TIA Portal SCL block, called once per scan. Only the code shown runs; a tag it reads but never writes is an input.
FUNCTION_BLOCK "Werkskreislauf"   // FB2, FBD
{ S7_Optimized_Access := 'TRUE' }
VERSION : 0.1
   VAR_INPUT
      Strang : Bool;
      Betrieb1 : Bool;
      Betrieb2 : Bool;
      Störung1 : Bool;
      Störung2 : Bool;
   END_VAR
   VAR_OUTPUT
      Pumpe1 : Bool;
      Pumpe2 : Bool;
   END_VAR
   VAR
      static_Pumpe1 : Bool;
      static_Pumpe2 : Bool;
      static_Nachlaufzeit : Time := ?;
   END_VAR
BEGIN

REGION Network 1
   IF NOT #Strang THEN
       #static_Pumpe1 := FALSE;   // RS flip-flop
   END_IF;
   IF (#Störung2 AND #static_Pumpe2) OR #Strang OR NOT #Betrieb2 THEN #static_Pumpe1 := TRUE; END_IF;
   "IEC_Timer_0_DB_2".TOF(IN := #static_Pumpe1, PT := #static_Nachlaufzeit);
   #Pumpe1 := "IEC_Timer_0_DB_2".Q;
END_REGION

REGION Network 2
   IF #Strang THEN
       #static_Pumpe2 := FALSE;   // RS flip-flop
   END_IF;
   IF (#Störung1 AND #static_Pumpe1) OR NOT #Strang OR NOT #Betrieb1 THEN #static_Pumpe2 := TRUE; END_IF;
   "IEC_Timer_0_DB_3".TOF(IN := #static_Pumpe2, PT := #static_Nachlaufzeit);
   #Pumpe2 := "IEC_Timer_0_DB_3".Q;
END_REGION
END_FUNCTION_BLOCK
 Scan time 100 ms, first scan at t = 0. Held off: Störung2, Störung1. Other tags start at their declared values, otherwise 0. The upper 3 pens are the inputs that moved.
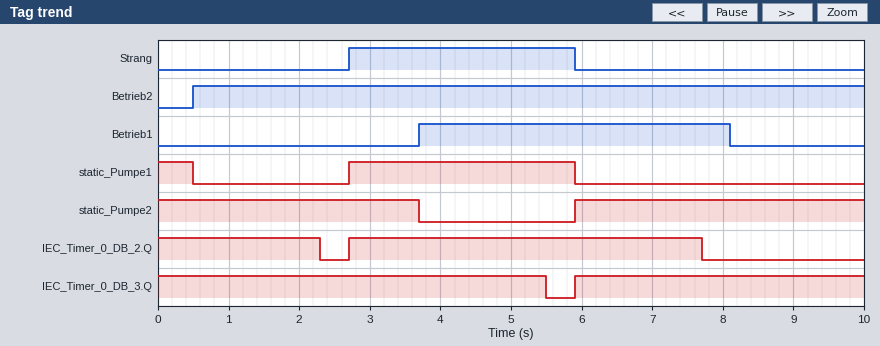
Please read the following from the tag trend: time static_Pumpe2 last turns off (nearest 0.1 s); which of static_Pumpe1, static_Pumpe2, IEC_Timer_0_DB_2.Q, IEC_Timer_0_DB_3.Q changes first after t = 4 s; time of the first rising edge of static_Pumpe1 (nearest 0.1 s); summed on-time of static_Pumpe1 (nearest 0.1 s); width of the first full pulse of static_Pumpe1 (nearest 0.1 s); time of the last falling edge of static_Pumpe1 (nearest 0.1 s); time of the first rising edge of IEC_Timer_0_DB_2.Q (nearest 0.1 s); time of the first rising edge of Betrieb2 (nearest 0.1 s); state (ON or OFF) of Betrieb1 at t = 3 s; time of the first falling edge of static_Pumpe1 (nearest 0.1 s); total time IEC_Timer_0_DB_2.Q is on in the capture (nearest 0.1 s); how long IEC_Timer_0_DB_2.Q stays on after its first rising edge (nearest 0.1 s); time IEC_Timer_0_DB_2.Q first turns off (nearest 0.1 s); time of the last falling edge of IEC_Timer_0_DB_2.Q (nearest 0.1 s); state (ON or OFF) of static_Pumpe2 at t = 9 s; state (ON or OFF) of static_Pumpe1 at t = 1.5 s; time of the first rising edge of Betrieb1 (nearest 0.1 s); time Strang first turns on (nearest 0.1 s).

3.7 s
IEC_Timer_0_DB_3.Q
2.7 s
3.7 s
3.2 s
5.9 s
2.7 s
0.5 s
OFF
0.5 s
7.3 s
5.0 s
2.3 s
7.7 s
ON
OFF
3.7 s
2.7 s
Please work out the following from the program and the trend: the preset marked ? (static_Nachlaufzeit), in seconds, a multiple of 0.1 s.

1.8 s
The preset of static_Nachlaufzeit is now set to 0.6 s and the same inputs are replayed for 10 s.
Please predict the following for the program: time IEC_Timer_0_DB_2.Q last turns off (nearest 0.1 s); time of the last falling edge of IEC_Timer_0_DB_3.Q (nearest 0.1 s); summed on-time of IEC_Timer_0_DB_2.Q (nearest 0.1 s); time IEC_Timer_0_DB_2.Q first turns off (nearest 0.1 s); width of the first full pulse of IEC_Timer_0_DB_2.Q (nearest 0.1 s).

6.5 s
4.3 s
4.9 s
1.1 s
3.8 s
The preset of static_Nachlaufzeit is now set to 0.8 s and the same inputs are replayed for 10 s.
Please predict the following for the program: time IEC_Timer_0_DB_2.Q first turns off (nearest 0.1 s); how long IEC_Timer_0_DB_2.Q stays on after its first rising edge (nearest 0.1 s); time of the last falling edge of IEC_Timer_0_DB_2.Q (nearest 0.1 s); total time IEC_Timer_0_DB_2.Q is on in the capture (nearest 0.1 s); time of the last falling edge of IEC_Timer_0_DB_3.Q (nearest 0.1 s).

1.3 s
4.0 s
6.7 s
5.3 s
4.5 s
